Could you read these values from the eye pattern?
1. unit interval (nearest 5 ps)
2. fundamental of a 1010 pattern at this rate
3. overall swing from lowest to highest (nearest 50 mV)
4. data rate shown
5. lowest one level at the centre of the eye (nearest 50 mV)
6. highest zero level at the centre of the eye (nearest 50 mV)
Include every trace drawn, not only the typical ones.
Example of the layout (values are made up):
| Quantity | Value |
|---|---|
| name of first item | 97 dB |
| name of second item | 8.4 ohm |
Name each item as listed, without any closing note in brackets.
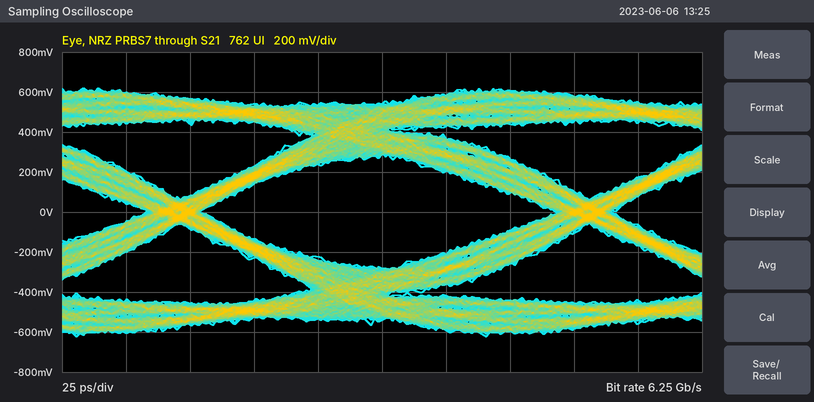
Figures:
| Quantity | Value |
|---|---|
| unit interval | 160 ps |
| fundamental of a 1010 pattern at this rate | 3.125 GHz |
| overall swing from lowest to highest | 1.25 V |
| data rate shown | 6.25 Gb/s |
| lowest one level at the centre of the eye | 300 mV |
| highest zero level at the centre of the eye | -300 mV |
